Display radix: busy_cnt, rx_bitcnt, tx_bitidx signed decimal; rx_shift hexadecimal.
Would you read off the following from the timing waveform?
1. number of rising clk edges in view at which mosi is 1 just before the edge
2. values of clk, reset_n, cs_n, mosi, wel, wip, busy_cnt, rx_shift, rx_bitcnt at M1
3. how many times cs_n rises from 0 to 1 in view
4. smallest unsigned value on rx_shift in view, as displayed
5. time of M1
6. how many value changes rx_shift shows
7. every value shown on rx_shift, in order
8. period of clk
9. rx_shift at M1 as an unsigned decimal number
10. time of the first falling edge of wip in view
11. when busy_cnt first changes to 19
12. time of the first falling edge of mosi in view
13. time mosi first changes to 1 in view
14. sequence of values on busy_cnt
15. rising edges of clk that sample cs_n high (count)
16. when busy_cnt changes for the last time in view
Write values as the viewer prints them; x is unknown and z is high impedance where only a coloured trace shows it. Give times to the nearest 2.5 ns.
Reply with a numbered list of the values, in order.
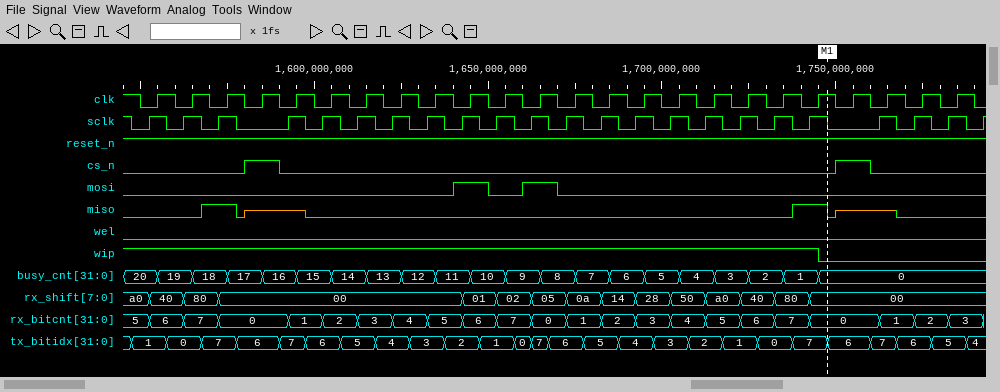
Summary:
1. 2
2. clk=1, reset_n=1, cs_n=0, mosi=0, wel=0, wip=0, busy_cnt=0, rx_shift=00, rx_bitcnt=0
3. 2
4. 00
5. 1747.5 ns
6. 14
7. a0, 40, 80, 00, 01, 02, 05, 0a, 14, 28, 50, a0, 40, 80, 00
8. 10 ns
9. 0
10. 1745 ns
11. 1555 ns
12. 1650 ns
13. 1640 ns
14. 20, 19, 18, 17, 16, 15, 14, 13, 12, 11, 10, 9, 8, 7, 6, 5, 4, 3, 2, 1, 0
15. 2
16. 1745 ns
